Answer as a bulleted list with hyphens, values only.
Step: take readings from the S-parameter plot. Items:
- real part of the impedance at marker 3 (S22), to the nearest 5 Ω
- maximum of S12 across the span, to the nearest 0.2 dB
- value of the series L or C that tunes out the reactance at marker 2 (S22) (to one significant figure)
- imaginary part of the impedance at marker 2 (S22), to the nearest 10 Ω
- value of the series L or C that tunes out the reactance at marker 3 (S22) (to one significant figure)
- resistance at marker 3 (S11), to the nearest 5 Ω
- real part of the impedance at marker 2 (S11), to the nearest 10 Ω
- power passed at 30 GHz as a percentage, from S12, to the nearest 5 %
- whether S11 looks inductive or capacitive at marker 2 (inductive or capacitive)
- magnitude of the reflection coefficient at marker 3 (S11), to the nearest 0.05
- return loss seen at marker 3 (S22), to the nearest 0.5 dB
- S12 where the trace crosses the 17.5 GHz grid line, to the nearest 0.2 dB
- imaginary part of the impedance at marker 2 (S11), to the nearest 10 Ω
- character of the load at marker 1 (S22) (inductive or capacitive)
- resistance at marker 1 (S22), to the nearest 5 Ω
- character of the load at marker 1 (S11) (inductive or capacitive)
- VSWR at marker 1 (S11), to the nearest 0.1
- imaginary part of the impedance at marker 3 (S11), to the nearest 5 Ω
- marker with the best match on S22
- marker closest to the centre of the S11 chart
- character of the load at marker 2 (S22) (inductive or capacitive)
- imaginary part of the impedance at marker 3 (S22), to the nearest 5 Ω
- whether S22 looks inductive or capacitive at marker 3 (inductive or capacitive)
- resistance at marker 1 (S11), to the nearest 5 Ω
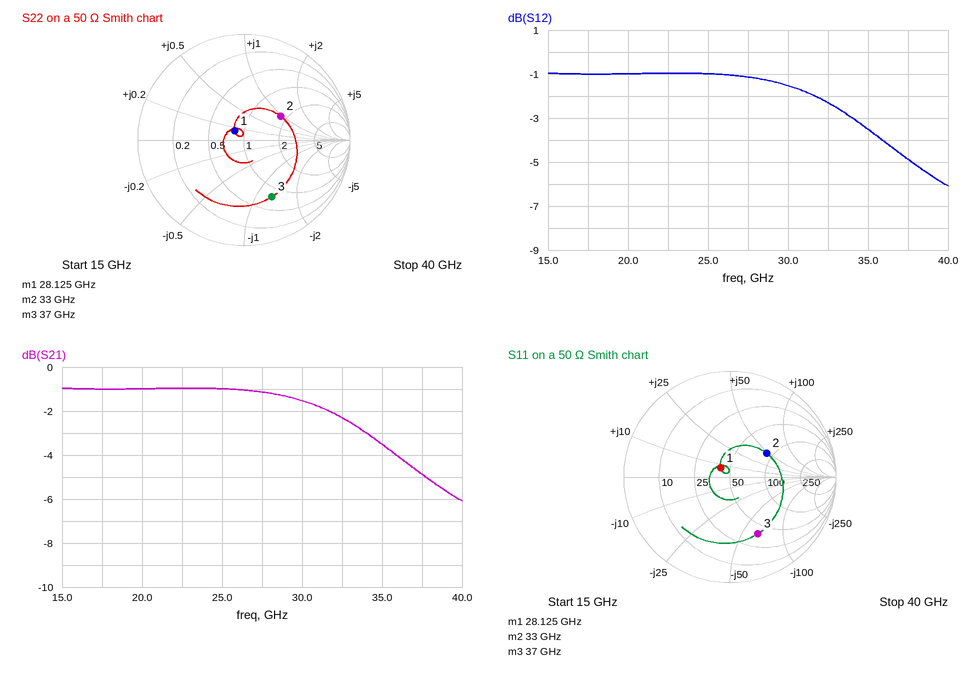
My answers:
- 40 Ω
- -1.0 dB
- 100 fF
- +50 Ω
- 300 pH
- 40 Ω
- 90 Ω
- 70 %
- inductive
- 0.60
- 4.5 dB
- -1.0 dB
- +50 Ω
- inductive
- 40 Ω
- inductive
- 1.3
- -65 Ω
- marker 1
- marker 1
- inductive
- -65 Ω
- capacitive
- 40 Ω
